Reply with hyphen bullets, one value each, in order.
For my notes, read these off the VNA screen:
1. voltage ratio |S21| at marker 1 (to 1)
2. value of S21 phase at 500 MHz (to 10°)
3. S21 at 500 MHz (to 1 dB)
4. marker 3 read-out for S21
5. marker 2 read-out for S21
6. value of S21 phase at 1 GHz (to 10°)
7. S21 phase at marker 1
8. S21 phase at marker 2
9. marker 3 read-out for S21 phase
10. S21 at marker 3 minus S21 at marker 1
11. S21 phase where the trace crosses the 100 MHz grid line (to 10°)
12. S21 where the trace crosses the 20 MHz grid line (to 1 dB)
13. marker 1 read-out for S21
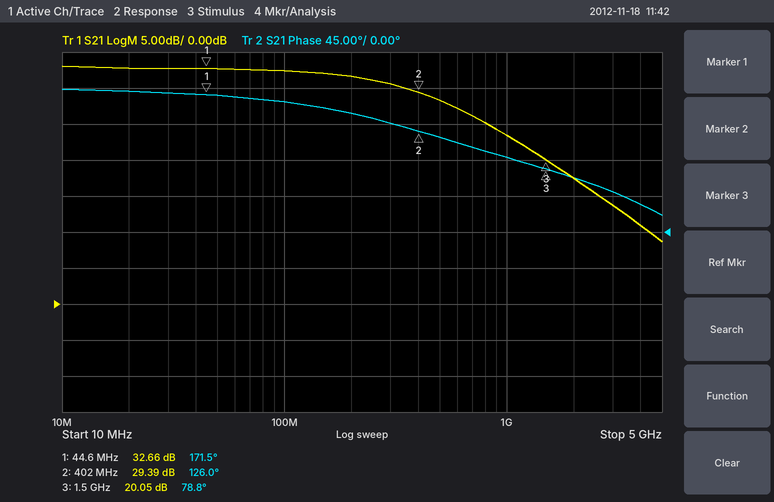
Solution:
- 43
- 120°
- 28 dB
- 20.05 dB
- 29.39 dB
- 90°
- 171.5°
- 126.0°
- 78.8°
- -12.61 dB
- 160°
- 33 dB
- 32.66 dB
